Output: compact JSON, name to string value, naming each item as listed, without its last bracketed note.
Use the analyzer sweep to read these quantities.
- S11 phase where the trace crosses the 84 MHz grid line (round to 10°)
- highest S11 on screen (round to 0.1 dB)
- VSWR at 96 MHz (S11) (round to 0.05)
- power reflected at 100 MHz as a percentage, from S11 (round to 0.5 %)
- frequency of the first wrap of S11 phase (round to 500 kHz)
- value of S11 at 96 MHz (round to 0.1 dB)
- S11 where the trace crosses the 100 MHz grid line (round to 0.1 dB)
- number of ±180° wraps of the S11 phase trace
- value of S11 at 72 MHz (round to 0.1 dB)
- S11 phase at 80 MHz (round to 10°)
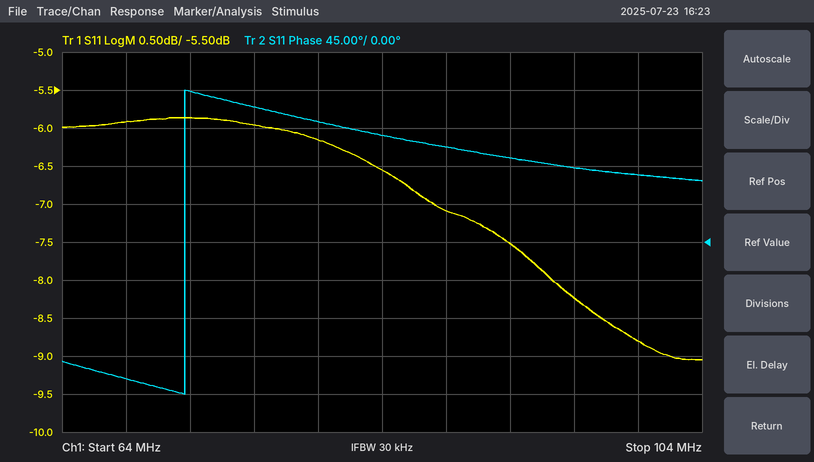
{"S11 phase where the trace crosses the 84 MHz grid line": "130°", "highest S11 on screen": "-5.9 dB", "VSWR at 96 MHz (S11)": "2.25", "power reflected at 100 MHz as a percentage, from S11": "13.0 %", "frequency of the first wrap of S11 phase": "71.5 MHz", "value of S11 at 96 MHz": "-8.2 dB", "S11 where the trace crosses the 100 MHz grid line": "-8.8 dB", "number of ±180° wraps of the S11 phase trace": "1", "value of S11 at 72 MHz": "-5.9 dB", "S11 phase at 80 MHz": "140°"}
